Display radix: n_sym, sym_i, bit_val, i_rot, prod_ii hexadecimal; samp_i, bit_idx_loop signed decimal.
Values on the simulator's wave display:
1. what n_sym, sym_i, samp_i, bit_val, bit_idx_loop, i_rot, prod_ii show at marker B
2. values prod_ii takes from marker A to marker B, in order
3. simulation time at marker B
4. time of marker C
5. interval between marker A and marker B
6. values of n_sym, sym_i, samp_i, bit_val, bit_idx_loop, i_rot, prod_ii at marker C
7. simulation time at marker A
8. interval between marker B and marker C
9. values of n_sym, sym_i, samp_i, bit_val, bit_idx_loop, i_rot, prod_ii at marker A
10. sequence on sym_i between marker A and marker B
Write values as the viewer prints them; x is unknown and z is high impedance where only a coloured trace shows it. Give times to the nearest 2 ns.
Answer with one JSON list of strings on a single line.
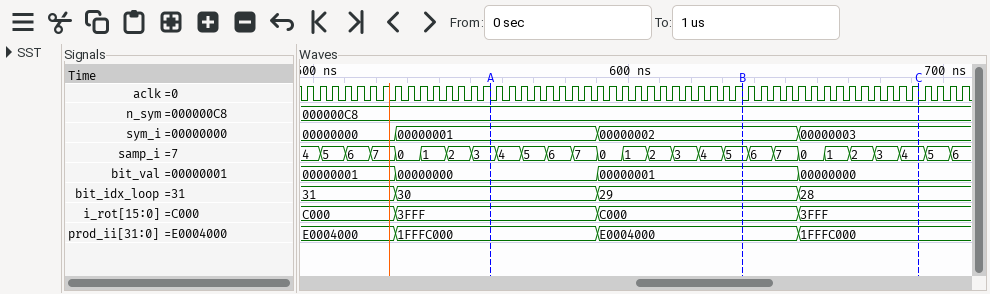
["n_sym=000000C8, sym_i=00000002, samp_i=5, bit_val=00000001, bit_idx_loop=29, i_rot=C000, prod_ii=E0004000", "1FFFC000, E0004000", "636 ns", "692 ns", "80 ns", "n_sym=000000C8, sym_i=00000003, samp_i=4, bit_val=00000000, bit_idx_loop=28, i_rot=3FFF, prod_ii=1FFFC000", "556 ns", "56 ns", "n_sym=000000C8, sym_i=00000001, samp_i=3, bit_val=00000000, bit_idx_loop=30, i_rot=3FFF, prod_ii=1FFFC000", "00000001, 00000002"]
